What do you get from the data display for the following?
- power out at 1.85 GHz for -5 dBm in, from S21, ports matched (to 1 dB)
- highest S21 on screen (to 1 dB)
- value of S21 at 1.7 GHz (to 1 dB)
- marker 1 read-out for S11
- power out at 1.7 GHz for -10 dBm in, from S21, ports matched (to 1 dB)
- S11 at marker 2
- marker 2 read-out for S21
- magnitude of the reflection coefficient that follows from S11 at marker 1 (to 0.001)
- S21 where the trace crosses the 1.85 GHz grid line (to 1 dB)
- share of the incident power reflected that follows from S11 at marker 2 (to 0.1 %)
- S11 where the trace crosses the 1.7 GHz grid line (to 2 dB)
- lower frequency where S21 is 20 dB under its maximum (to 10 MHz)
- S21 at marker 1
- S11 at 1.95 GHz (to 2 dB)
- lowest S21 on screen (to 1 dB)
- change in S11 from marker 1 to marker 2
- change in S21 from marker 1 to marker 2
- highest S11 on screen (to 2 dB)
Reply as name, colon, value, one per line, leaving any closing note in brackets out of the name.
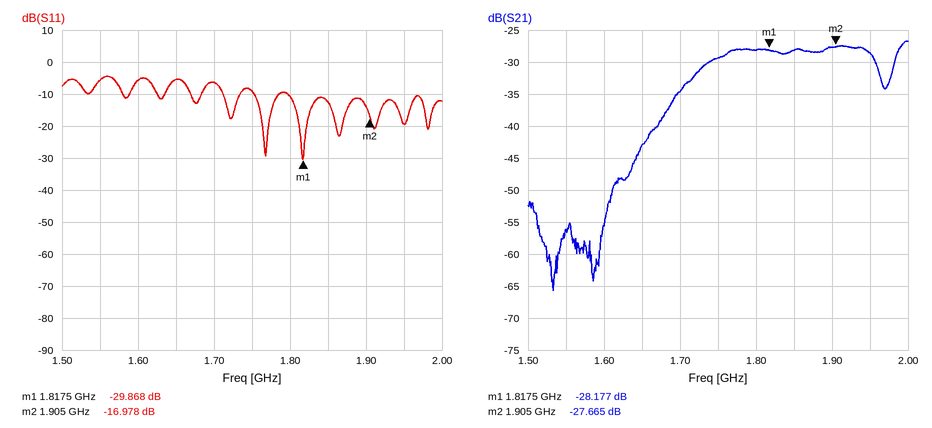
power out at 1.85 GHz for -5 dBm in, from S21, ports matched: -33 dBm
highest S21 on screen: -27 dB
value of S21 at 1.7 GHz: -35 dB
marker 1 read-out for S11: -29.868 dB
power out at 1.7 GHz for -10 dBm in, from S21, ports matched: -45 dBm
S11 at marker 2: -16.978 dB
marker 2 read-out for S21: -27.665 dB
magnitude of the reflection coefficient that follows from S11 at marker 1: 0.032
S21 where the trace crosses the 1.85 GHz grid line: -28 dB
share of the incident power reflected that follows from S11 at marker 2: 2.0 %
S11 where the trace crosses the 1.7 GHz grid line: -6 dB
lower frequency where S21 is 20 dB under its maximum: 1.64 GHz
S21 at marker 1: -28.177 dB
S11 at 1.95 GHz: -20 dB
lowest S21 on screen: -66 dB
change in S11 from marker 1 to marker 2: 12.890 dB
change in S21 from marker 1 to marker 2: 0.512 dB
highest S11 on screen: -4 dB
